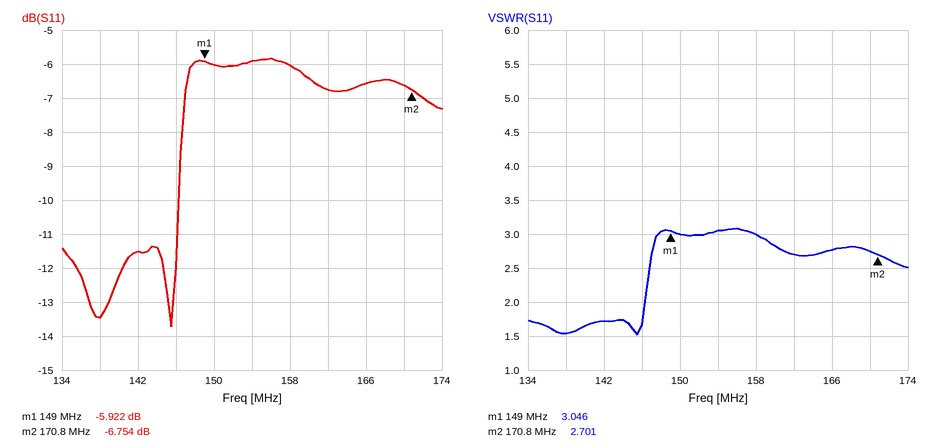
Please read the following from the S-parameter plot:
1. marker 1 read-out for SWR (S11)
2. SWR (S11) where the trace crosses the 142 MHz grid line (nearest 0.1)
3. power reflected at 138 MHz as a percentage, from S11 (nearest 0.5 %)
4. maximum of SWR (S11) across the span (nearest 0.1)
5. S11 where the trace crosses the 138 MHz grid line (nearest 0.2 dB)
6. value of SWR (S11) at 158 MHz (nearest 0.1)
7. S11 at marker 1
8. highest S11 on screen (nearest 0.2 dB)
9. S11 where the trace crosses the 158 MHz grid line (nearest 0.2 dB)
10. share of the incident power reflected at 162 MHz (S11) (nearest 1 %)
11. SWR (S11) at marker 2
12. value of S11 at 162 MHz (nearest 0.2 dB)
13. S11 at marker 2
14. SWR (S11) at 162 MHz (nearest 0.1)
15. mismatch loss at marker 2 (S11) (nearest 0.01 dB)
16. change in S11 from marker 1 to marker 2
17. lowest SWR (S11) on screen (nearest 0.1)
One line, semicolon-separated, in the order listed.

3.046; 1.7; 4.5 %; 3.1; -13.4 dB; 3.0; -5.922 dB; -5.8 dB; -6.0 dB; 21 %; 2.701; -6.8 dB; -6.754 dB; 2.7; 1.03 dB; -0.832 dB; 1.5
